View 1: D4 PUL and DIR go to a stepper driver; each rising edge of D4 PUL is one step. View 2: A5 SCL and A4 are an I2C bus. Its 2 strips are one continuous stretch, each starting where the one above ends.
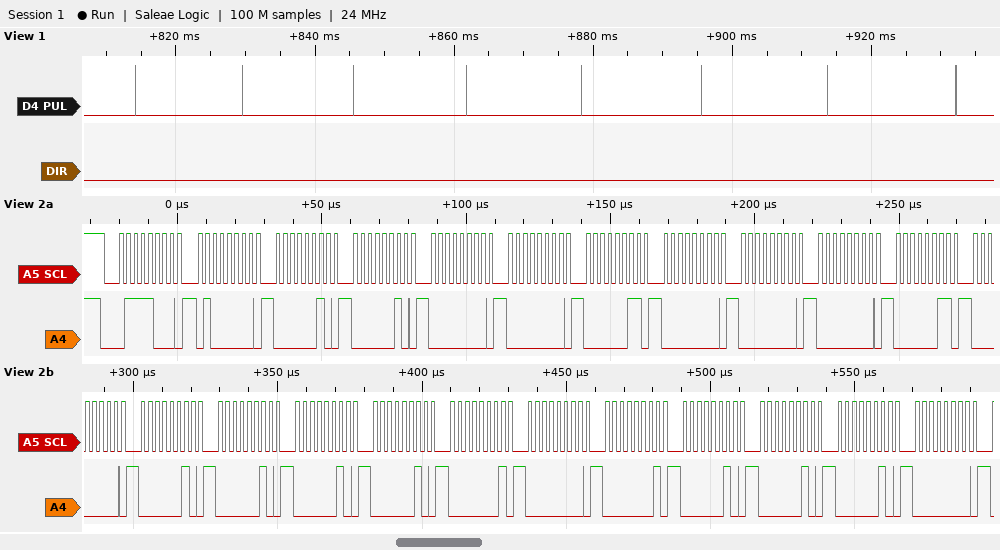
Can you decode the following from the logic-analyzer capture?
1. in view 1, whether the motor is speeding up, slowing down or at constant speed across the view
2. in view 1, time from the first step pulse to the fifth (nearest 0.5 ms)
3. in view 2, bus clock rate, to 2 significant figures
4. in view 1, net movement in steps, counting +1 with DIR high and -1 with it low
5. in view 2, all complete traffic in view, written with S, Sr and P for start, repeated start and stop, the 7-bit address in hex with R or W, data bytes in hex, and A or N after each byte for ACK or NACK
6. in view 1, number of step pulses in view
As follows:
slowing down
64.0 ms
400 kHz
-8
S 3CW A 40 A 02 A 02 A 00 A 00 A 03 A 00 A 00 A 00 A 03 A 00 A 02 A 02 A 02 A 02 A 01 A 00 A 01 A 02 A 02 A 02 A 00 A
8
